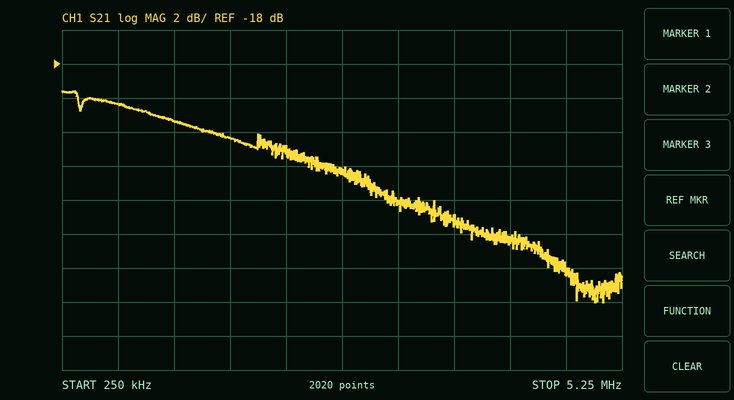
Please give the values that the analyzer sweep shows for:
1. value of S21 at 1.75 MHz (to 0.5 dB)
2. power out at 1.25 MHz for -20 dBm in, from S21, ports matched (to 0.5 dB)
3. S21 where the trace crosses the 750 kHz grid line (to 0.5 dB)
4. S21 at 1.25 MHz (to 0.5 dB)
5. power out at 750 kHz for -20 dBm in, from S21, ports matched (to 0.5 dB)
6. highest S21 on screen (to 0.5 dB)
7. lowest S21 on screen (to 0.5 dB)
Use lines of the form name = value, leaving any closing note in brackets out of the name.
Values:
value of S21 at 1.75 MHz = -22.5 dB
power out at 1.25 MHz for -20 dBm in, from S21, ports matched = -41.5 dBm
S21 where the trace crosses the 750 kHz grid line = -20.5 dB
S21 at 1.25 MHz = -21.5 dB
power out at 750 kHz for -20 dBm in, from S21, ports matched = -40.5 dBm
highest S21 on screen = -19.5 dB
lowest S21 on screen = -32.0 dB
